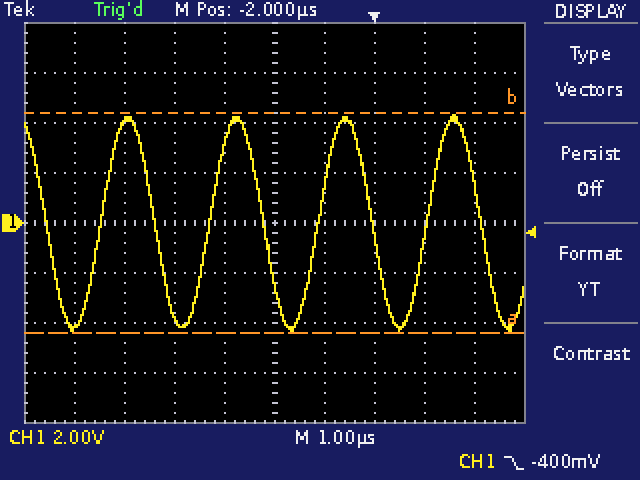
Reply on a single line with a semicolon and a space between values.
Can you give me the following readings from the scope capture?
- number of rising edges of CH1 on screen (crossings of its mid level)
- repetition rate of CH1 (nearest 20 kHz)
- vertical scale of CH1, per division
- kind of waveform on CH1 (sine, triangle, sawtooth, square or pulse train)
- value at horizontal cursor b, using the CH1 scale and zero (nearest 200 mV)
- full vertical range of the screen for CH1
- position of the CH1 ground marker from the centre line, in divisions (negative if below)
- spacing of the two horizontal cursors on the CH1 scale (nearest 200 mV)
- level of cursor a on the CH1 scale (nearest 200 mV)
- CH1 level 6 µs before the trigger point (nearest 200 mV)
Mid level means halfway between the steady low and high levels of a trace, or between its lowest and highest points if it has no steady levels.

4; 460 kHz; 2 V; sine; 4.4 V; 16 V; 0.0 div; 8.8 V; -4.4 V; -4.2 V
